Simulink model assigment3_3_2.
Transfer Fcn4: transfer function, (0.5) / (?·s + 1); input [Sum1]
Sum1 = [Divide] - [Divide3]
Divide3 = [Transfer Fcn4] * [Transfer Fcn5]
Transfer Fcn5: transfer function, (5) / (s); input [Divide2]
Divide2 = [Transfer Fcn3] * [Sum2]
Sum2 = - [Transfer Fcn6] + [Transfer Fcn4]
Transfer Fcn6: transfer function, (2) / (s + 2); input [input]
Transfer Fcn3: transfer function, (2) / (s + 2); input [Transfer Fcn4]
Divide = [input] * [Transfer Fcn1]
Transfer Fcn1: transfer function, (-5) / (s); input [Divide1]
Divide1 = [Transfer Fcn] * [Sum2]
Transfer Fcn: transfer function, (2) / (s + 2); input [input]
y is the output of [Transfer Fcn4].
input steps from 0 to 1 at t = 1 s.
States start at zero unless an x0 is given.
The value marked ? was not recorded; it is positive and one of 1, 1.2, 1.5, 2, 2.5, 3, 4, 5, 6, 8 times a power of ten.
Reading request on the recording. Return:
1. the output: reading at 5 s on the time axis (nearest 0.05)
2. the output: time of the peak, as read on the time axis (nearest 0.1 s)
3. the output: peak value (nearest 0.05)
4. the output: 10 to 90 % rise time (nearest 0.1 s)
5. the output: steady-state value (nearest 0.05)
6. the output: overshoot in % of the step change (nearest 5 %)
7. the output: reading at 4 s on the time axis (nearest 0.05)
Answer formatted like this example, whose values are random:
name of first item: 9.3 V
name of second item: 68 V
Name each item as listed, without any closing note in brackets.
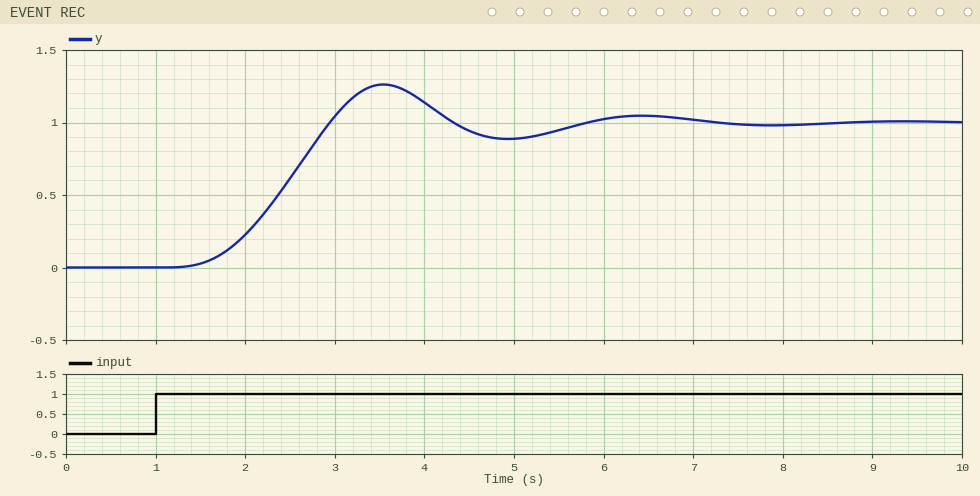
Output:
the output: reading at 5 s on the time axis: 0.90
the output: time of the peak, as read on the time axis: 3.5 s
the output: peak value: 1.25
the output: 10 to 90 % rise time: 1.1 s
the output: steady-state value: 1.00
the output: overshoot in % of the step change: 25 %
the output: reading at 4 s on the time axis: 1.15
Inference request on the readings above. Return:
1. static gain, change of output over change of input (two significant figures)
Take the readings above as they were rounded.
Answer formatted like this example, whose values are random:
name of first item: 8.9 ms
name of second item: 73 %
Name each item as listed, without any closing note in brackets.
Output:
static gain, change of output over change of input: 1.0
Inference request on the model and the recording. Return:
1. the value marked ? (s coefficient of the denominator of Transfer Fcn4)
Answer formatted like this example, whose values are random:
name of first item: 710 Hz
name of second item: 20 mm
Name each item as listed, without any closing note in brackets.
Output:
the value marked ?: 1
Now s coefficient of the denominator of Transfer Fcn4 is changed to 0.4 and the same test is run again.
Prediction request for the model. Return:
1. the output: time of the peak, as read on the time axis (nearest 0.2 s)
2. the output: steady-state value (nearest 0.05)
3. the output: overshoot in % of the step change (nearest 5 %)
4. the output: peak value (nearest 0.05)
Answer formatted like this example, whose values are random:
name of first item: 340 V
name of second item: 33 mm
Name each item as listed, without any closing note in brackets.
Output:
the output: time of the peak, as read on the time axis: 3.0 s
the output: steady-state value: 1.00
the output: overshoot in % of the step change: 10 %
the output: peak value: 1.10
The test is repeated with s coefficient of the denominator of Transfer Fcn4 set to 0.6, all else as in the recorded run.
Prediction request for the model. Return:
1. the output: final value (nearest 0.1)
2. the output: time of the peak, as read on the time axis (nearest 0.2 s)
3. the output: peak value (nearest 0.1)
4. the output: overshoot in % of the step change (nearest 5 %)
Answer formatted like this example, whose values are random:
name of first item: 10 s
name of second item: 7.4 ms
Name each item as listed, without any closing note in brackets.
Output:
the output: final value: 1.0
the output: time of the peak, as read on the time axis: 3.2 s
the output: peak value: 1.2
the output: overshoot in % of the step change: 15 %
